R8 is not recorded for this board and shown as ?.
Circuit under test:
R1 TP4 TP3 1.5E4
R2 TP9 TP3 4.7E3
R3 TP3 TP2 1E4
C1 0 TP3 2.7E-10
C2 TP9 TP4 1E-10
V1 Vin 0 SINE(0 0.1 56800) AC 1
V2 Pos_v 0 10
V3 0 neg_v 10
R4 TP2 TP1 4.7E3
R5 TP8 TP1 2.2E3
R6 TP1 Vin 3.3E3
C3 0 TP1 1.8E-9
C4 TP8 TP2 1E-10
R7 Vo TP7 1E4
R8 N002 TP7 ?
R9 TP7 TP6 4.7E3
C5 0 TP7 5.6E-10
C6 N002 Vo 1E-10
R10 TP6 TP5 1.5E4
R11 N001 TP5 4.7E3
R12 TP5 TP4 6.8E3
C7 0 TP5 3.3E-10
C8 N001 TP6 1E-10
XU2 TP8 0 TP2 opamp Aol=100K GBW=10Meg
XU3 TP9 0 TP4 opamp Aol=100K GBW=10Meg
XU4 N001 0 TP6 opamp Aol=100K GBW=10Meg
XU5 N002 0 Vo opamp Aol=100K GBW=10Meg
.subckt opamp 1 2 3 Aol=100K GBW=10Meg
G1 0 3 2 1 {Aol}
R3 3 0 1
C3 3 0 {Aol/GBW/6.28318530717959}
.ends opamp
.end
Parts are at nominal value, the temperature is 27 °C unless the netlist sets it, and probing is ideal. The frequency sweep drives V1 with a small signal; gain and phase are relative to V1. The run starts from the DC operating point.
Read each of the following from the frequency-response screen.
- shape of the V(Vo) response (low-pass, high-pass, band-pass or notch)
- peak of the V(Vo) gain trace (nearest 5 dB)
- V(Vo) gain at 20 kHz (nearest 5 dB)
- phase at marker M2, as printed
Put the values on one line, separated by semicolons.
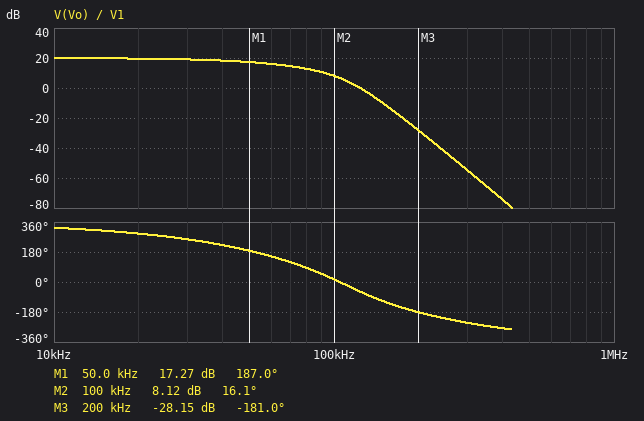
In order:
low-pass; 20 dB; 20 dB; 16.1 deg
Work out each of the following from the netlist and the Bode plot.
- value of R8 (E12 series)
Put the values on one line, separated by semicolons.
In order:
5.6 kΩ
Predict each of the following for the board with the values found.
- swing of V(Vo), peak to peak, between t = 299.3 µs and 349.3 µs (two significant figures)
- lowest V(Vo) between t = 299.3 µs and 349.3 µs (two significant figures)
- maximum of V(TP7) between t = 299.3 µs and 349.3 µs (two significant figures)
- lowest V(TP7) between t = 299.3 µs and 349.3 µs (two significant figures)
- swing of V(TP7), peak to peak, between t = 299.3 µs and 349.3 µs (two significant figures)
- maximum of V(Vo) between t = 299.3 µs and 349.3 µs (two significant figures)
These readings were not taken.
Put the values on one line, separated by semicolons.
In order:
1.3 V; -660 mV; 140 mV; -140 mV; 270 mV; 660 mV
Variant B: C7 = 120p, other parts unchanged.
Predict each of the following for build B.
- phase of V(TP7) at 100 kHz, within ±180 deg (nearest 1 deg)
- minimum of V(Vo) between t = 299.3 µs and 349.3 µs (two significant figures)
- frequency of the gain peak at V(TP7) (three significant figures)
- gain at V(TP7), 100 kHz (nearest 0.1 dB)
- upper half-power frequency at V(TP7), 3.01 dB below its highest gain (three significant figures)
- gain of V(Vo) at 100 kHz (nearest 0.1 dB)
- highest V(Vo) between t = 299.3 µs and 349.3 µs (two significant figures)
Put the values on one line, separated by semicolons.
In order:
-56 deg; -610 mV; 60.6 kHz; -1.2 dB; 99.0 kHz; 7.6 dB; 610 mV
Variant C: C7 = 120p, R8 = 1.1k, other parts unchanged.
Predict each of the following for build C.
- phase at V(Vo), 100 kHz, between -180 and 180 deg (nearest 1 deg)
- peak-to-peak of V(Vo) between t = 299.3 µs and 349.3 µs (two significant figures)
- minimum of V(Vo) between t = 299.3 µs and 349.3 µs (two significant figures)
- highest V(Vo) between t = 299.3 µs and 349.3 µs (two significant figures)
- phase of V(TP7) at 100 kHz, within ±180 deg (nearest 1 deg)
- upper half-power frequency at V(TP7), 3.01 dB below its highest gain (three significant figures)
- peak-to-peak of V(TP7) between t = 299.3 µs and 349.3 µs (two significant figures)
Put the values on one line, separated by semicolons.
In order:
82 deg; 1.4 V; -680 mV; 680 mV; -7 deg; 115 kHz; 61 mV
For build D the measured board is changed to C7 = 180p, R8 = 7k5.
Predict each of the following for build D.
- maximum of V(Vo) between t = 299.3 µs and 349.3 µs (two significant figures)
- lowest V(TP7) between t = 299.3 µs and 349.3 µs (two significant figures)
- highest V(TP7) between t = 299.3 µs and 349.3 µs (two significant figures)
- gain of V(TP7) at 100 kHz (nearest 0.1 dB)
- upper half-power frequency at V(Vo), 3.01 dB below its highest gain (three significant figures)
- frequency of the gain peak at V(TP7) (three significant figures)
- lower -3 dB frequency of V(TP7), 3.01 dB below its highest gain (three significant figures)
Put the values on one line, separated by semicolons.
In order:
560 mV; -150 mV; 150 mV; -0.5 dB; 43.2 kHz; 54.4 kHz; 25.5 kHz
